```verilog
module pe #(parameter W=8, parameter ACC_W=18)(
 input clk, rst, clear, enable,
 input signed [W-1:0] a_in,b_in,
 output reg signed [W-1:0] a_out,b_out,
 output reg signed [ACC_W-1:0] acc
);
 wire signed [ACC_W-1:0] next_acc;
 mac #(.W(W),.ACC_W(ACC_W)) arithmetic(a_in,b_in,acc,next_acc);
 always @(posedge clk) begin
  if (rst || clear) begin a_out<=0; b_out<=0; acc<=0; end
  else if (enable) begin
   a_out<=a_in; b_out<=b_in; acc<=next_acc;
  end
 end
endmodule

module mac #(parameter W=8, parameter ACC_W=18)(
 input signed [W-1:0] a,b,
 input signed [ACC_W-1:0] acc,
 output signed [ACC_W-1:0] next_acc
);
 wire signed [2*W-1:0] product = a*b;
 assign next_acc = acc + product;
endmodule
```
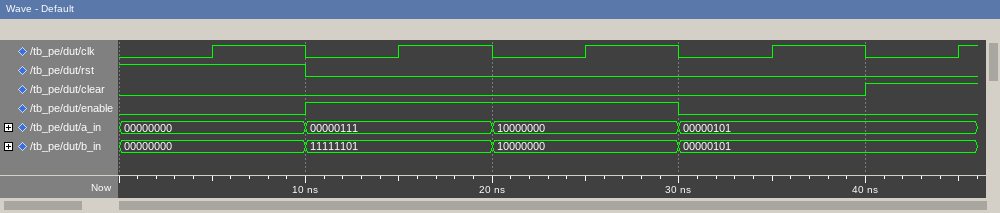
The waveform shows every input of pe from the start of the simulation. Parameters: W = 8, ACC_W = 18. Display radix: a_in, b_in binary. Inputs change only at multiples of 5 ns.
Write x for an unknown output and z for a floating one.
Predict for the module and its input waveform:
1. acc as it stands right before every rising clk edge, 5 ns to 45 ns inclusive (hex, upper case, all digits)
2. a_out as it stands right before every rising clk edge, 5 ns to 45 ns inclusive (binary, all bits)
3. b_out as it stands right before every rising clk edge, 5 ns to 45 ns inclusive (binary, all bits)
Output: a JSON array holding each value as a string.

["x, 00000, 3FFEB, 03FEB, 03FEB", "x, 00000000, 00000111, 10000000, 10000000", "x, 00000000, 11111101, 10000000, 10000000"]
